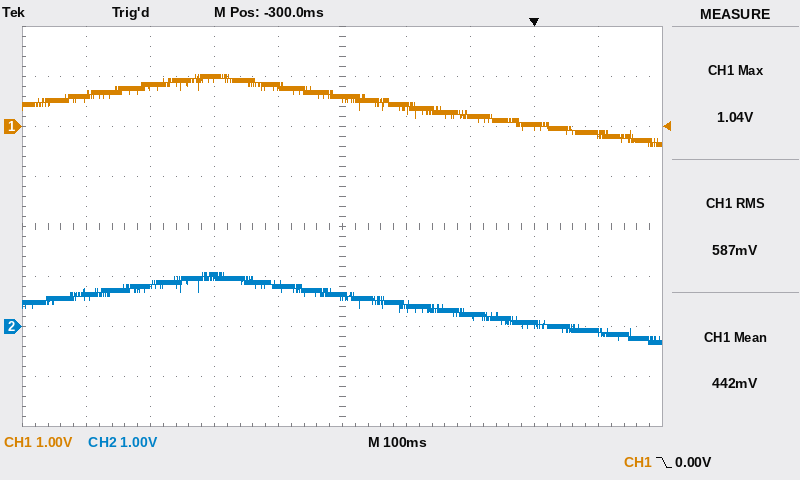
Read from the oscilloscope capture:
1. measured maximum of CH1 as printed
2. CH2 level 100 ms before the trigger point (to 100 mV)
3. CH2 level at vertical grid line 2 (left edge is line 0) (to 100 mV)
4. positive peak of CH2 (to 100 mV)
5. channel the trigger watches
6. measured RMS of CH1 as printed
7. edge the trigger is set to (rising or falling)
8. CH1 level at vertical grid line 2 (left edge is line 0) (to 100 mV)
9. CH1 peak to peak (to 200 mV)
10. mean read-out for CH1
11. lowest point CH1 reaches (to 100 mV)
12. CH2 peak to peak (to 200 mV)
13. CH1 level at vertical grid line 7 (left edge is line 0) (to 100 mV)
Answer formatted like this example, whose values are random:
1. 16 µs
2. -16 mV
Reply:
1. 1.04 V
2. 200 mV
3. 800 mV
4. 1.1 V
5. CH1
6. 587 mV
7. falling
8. 800 mV
9. 1.4 V
10. 442 mV
11. -400 mV
12. 1.4 V
13. 200 mV
